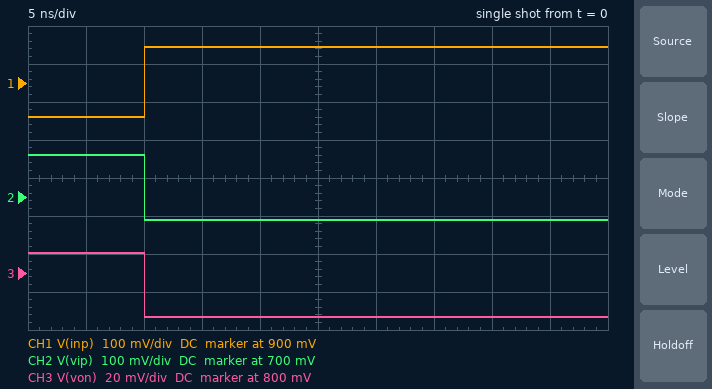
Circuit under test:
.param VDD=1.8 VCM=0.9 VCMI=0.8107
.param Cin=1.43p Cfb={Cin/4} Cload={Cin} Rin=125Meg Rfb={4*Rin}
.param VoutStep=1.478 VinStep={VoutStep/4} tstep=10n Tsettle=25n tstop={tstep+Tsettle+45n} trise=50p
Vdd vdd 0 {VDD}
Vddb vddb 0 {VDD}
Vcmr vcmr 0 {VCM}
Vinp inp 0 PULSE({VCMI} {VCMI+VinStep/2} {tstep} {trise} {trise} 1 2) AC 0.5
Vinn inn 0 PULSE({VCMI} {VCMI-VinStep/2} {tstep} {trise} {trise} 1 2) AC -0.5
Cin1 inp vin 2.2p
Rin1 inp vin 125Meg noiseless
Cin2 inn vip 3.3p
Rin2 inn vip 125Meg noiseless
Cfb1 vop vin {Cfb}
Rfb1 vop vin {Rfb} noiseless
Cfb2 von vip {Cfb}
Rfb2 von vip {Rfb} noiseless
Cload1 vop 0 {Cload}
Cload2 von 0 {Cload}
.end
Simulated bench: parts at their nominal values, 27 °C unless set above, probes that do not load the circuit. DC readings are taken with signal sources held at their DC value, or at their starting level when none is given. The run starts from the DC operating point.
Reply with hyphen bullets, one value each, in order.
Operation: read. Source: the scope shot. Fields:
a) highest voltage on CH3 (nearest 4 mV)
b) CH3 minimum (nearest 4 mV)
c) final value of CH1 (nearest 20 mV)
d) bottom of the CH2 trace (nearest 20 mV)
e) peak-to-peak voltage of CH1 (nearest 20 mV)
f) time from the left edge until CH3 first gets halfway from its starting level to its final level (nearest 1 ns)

- 812 mV
- 776 mV
- 1.00 V
- 640 mV
- 180 mV
- 10 ns
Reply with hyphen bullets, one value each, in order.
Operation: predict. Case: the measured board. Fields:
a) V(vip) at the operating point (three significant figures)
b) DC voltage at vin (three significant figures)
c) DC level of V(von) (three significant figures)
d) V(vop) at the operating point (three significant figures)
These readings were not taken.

- 811 mV
- 811 mV
- 811 mV
- 811 mV
